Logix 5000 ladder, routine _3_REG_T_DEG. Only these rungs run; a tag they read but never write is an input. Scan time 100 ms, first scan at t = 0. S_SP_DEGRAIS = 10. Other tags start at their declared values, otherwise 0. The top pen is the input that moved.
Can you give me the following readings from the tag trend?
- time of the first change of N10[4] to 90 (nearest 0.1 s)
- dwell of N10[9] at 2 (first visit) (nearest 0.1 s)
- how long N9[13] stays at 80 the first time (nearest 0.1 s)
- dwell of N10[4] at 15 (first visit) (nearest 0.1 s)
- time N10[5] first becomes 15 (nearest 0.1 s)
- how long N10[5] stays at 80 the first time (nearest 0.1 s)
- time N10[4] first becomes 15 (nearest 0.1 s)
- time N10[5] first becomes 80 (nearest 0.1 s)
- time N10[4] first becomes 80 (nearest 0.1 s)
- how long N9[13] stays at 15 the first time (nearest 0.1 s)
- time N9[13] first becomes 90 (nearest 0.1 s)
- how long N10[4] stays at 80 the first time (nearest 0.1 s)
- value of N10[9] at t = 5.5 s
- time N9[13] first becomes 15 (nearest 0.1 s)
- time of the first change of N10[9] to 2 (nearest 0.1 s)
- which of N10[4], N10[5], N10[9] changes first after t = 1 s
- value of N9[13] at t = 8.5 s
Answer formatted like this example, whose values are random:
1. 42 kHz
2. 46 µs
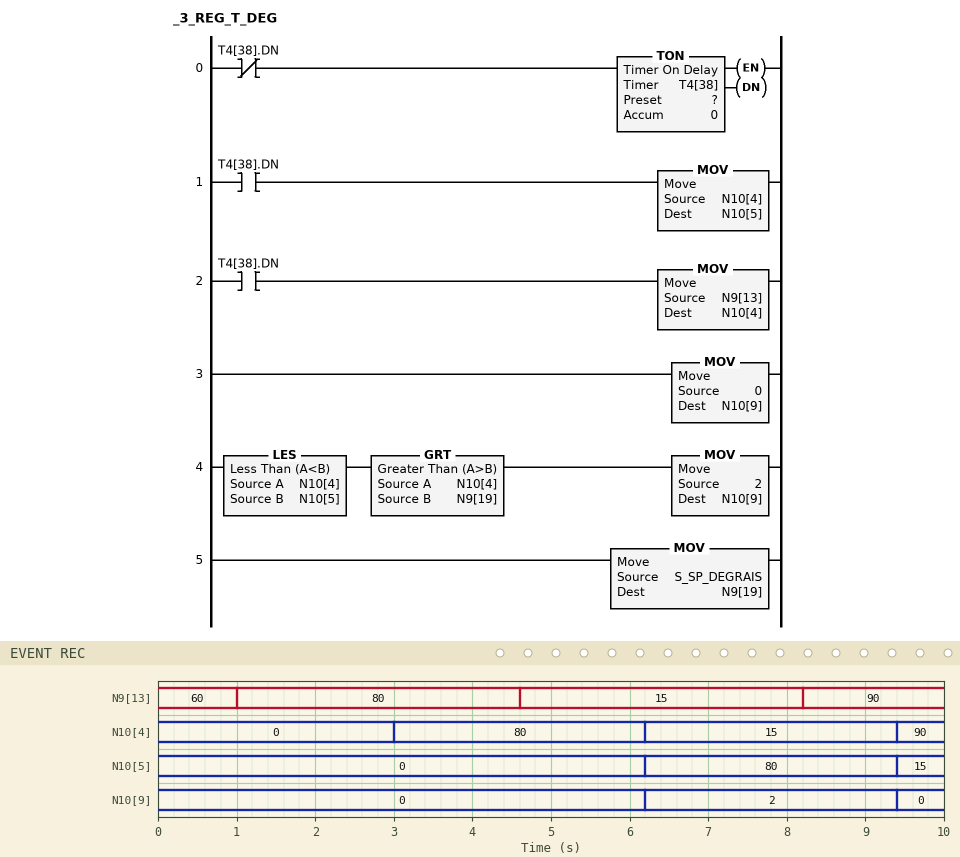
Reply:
1. 9.4 s
2. 3.2 s
3. 3.6 s
4. 3.2 s
5. 9.4 s
6. 3.2 s
7. 6.2 s
8. 6.2 s
9. 3.0 s
10. 3.6 s
11. 8.2 s
12. 3.2 s
13. 0
14. 4.6 s
15. 6.2 s
16. N10[4]
17. 90
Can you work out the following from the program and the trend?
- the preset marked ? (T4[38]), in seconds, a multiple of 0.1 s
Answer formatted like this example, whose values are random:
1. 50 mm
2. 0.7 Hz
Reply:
1. 3.0 s
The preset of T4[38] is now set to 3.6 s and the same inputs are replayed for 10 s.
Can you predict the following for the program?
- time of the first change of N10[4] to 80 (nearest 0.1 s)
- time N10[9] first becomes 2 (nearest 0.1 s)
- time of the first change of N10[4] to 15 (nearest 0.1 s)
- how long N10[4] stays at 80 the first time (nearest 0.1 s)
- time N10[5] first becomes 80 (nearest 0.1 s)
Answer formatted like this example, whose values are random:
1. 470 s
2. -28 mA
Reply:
1. 3.6 s
2. 7.4 s
3. 7.4 s
4. 3.8 s
5. 7.4 s
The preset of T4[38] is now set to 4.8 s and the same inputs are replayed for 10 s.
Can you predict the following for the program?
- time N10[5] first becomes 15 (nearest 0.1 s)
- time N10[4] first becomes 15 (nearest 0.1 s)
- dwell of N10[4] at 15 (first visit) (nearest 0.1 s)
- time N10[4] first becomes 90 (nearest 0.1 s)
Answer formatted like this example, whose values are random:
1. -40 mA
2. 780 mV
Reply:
1. 9.8 s
2. 4.8 s
3. 5.0 s
4. 9.8 s
